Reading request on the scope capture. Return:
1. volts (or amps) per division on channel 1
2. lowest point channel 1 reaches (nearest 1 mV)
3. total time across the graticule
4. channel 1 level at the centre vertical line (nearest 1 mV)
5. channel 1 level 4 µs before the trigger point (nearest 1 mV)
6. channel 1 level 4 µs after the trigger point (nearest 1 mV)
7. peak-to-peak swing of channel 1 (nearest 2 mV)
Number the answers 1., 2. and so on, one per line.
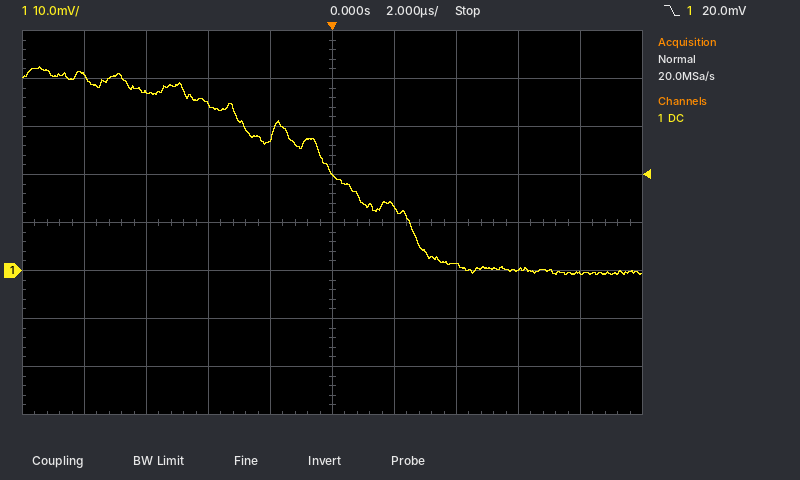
1. 10 mV
2. -1 mV
3. 20 µs
4. 20 mV
5. 35 mV
6. 1 mV
7. 44 mV
